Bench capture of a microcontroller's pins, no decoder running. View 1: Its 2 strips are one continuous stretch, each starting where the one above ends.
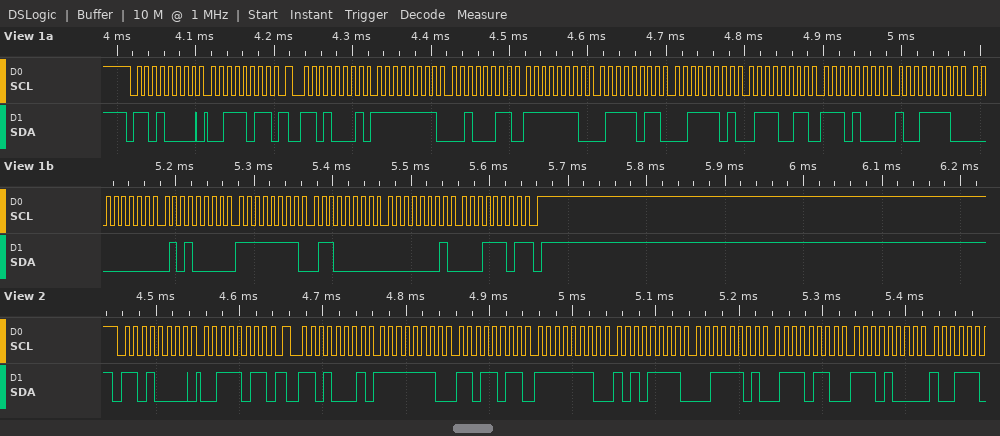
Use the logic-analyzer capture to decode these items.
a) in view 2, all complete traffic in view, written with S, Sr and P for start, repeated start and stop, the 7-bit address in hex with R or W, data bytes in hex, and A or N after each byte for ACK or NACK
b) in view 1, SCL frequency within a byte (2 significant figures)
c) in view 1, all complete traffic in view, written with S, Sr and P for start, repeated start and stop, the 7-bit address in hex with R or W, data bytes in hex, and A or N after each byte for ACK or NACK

S 68W A 3B A Sr 68R A FE A DB A FE A AF A 3D A 76 A E8 A
100 kHz
S 68W A 3B A Sr 68R A FF A 23 A FE A 7B A 3D A 73 A E8 A 9E A 00 A 50 A FF A 60 A 01 A 1D N P
